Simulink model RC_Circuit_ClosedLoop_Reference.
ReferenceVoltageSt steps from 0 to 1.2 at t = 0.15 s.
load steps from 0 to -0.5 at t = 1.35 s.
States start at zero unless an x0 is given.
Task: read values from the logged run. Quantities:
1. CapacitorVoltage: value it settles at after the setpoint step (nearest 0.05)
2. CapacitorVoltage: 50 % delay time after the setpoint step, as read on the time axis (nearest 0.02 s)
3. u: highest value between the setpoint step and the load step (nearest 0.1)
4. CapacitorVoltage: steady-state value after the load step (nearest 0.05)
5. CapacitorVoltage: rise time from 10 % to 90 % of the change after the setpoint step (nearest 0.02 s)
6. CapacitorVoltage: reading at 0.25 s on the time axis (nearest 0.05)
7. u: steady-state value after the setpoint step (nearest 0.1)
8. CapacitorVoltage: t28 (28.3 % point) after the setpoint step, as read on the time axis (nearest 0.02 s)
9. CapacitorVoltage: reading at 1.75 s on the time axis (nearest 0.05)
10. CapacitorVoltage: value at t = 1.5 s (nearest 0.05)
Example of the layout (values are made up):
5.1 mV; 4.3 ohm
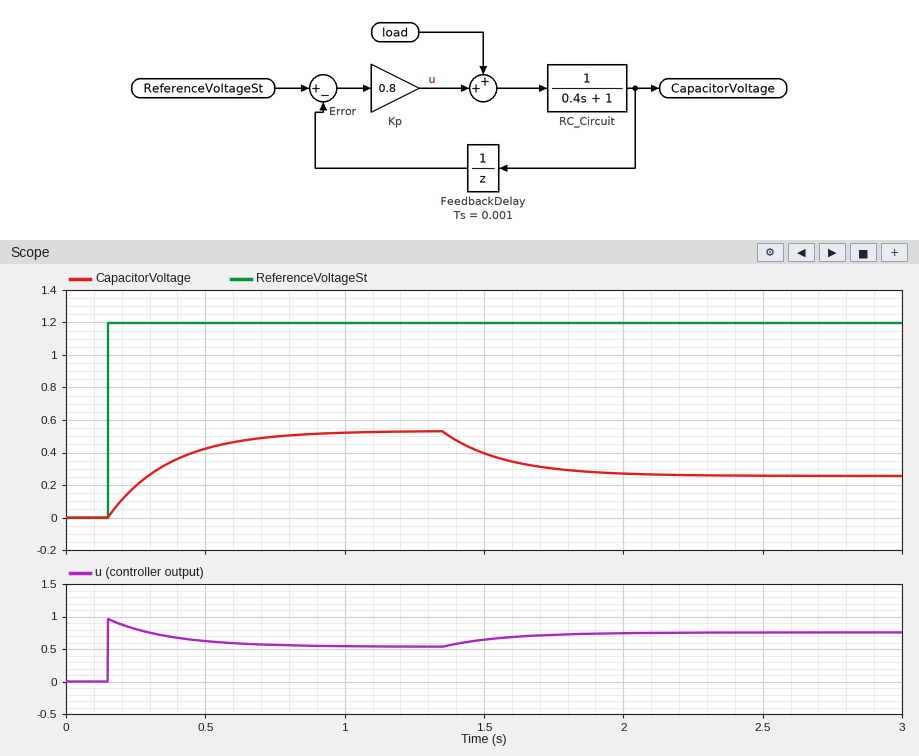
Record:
0.55; 0.30 s; 1.0; 0.25; 0.48 s; 0.20; 0.5; 0.22 s; 0.30; 0.40
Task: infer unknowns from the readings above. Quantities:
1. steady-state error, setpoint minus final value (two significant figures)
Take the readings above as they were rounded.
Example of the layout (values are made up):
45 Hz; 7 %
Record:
0.65
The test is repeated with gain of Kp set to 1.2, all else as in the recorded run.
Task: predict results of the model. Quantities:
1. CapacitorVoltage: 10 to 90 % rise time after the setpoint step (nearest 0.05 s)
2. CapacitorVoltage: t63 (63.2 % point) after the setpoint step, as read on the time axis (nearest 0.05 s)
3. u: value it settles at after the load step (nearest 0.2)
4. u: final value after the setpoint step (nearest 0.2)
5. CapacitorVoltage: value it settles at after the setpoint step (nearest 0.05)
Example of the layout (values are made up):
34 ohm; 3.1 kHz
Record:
0.40 s; 0.35 s; 1.0; 0.6; 0.65
